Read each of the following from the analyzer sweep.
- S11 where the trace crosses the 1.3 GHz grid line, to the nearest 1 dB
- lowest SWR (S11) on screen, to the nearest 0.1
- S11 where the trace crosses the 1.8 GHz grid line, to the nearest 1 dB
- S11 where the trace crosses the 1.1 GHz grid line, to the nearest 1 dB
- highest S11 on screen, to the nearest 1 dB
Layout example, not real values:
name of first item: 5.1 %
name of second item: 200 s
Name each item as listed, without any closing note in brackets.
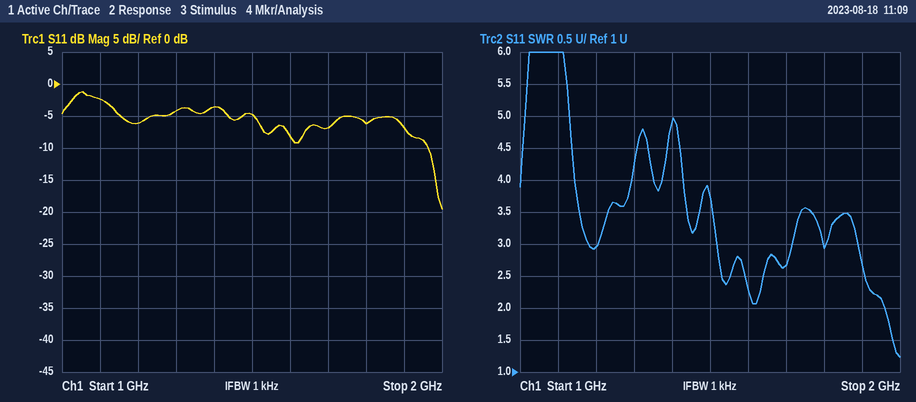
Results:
S11 where the trace crosses the 1.3 GHz grid line, to the nearest 1 dB: -4 dB
lowest SWR (S11) on screen, to the nearest 0.1: 1.2
S11 where the trace crosses the 1.8 GHz grid line, to the nearest 1 dB: -6 dB
S11 where the trace crosses the 1.1 GHz grid line, to the nearest 1 dB: -2 dB
highest S11 on screen, to the nearest 1 dB: -1 dB
